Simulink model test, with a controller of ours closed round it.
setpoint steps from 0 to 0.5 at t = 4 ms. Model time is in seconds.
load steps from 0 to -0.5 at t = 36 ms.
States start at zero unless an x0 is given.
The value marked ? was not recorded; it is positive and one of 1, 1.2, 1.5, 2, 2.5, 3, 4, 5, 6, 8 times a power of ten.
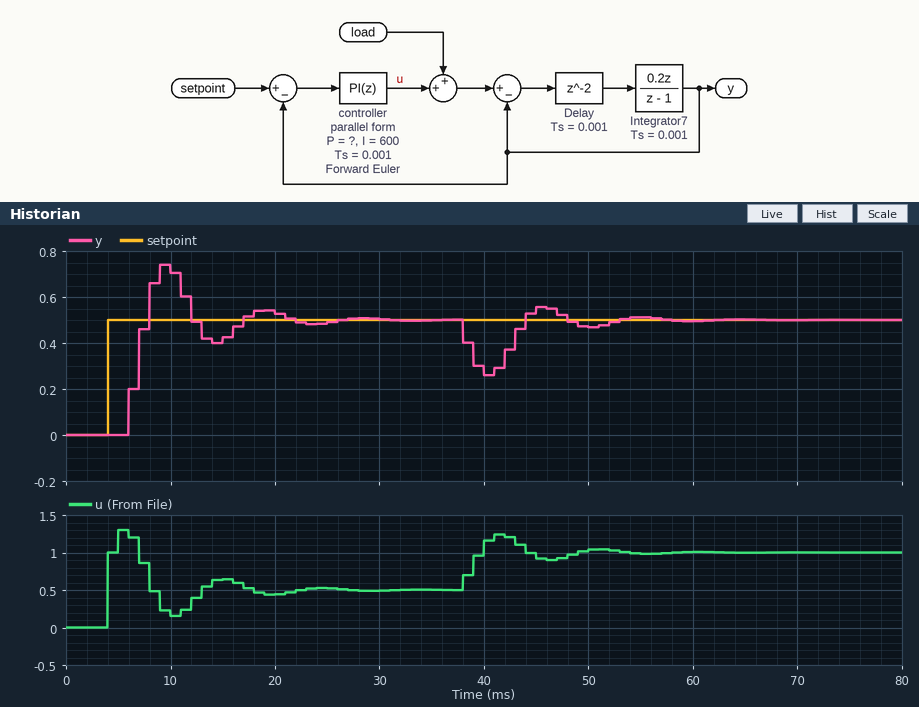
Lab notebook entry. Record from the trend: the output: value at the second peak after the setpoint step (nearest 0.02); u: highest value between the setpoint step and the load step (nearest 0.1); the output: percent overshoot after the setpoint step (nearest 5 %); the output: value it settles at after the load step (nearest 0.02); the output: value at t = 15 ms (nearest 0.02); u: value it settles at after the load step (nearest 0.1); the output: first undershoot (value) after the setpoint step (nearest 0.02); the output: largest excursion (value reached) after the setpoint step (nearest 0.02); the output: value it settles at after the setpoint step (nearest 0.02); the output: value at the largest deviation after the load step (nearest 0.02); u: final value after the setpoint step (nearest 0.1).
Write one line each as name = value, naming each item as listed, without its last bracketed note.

the output: value at the second peak after the setpoint step = 0.54
u: highest value between the setpoint step and the load step = 1.3
the output: percent overshoot after the setpoint step = 50 %
the output: value it settles at after the load step = 0.50
the output: value at t = 15 ms = 0.42
u: value it settles at after the load step = 1.0
the output: first undershoot (value) after the setpoint step = 0.40
the output: largest excursion (value reached) after the setpoint step = 0.74
the output: value it settles at after the setpoint step = 0.50
the output: value at the largest deviation after the load step = 0.26
u: final value after the setpoint step = 0.5
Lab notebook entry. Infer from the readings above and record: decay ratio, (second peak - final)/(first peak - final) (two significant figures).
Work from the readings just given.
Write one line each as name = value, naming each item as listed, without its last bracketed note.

decay ratio, (second peak - final)/(first peak - final) = 0.17
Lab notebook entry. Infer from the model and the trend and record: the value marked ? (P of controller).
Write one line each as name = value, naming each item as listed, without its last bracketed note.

the value marked ? = 2
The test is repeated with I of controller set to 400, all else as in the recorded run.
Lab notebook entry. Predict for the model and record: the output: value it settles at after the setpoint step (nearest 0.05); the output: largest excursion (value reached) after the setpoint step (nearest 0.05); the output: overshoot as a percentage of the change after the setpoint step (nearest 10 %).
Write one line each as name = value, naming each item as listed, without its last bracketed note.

the output: value it settles at after the setpoint step = 0.50
the output: largest excursion (value reached) after the setpoint step = 0.65
the output: overshoot as a percentage of the change after the setpoint step = 30 %
